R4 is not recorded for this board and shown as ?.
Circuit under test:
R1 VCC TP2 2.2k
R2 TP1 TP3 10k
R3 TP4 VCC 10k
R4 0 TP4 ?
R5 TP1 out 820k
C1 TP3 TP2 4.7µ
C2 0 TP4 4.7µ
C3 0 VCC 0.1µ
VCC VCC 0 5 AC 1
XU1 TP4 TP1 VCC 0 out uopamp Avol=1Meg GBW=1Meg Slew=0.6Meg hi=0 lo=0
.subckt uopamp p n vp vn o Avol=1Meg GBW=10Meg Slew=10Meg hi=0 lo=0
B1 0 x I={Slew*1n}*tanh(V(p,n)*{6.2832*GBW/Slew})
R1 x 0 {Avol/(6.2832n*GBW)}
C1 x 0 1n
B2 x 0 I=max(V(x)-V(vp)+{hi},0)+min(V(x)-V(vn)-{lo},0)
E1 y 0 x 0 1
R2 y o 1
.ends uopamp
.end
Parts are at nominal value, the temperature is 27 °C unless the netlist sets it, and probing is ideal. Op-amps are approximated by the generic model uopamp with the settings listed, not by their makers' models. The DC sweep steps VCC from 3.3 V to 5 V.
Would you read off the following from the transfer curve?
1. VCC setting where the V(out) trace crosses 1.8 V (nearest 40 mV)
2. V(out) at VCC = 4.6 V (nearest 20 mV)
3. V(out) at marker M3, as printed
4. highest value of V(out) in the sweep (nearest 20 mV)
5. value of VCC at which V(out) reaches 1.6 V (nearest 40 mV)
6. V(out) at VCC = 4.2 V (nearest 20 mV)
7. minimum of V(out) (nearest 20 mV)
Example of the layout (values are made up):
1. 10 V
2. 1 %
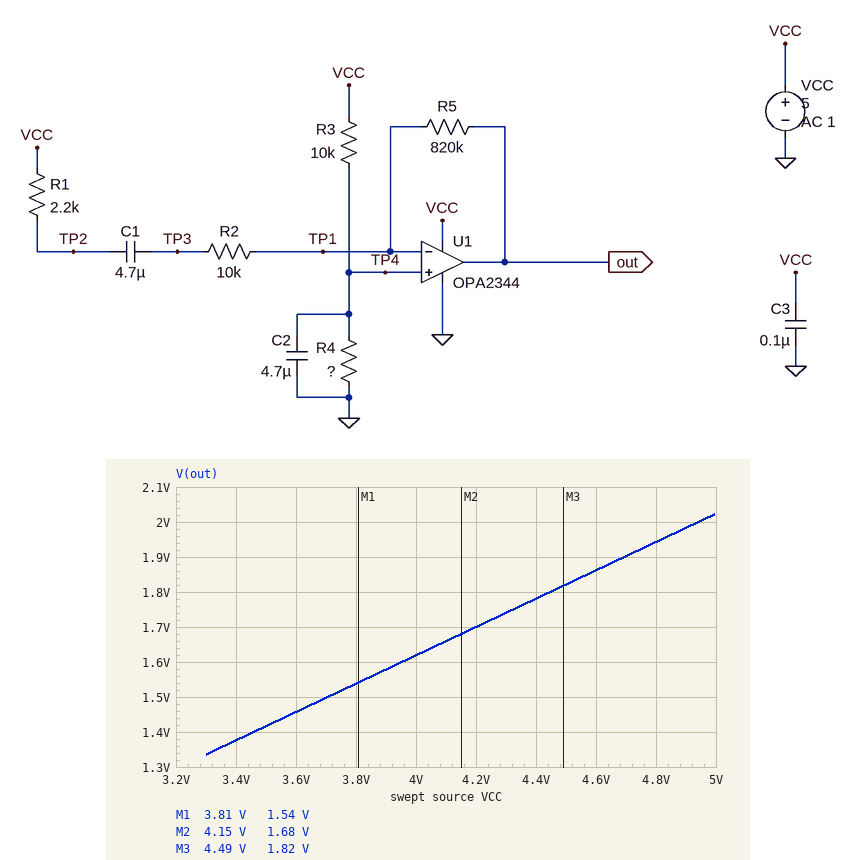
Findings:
1. 4.44 V
2. 1.86 V
3. 1.82 V
4. 2.02 V
5. 3.96 V
6. 1.70 V
7. 1.34 V
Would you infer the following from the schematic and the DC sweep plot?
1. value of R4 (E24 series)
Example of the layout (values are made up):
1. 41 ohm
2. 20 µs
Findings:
1. 6.8 kΩ
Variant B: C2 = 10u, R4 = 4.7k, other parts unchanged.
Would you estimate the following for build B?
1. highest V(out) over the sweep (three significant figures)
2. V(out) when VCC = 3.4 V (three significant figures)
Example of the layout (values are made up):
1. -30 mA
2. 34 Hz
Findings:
1. 1.60 V
2. 1.09 V
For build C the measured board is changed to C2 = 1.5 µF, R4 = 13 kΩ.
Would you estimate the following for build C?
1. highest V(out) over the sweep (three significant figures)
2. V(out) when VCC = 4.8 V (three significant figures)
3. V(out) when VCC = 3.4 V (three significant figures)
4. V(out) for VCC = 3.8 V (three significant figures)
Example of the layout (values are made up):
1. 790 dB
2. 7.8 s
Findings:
1. 2.83 V
2. 2.71 V
3. 1.92 V
4. 2.15 V
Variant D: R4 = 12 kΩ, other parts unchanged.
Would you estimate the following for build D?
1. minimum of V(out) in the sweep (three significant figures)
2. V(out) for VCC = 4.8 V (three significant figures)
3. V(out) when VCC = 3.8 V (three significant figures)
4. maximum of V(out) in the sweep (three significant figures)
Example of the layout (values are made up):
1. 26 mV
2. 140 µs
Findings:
1. 1.80 V
2. 2.62 V
3. 2.07 V
4. 2.73 V
